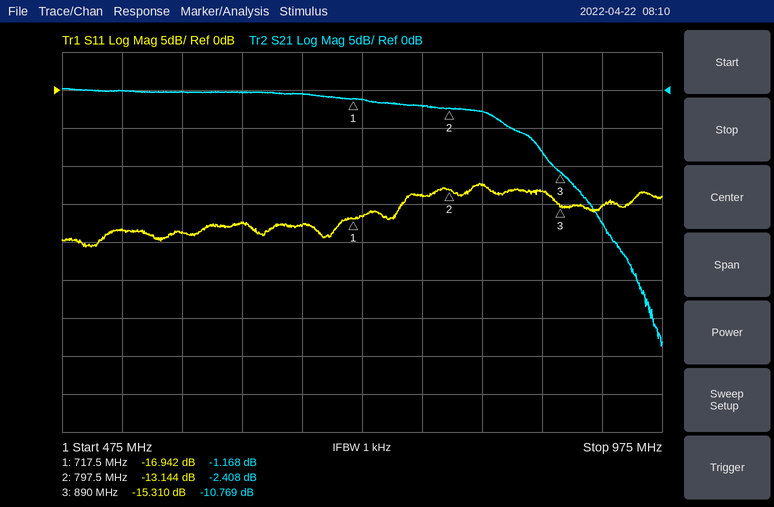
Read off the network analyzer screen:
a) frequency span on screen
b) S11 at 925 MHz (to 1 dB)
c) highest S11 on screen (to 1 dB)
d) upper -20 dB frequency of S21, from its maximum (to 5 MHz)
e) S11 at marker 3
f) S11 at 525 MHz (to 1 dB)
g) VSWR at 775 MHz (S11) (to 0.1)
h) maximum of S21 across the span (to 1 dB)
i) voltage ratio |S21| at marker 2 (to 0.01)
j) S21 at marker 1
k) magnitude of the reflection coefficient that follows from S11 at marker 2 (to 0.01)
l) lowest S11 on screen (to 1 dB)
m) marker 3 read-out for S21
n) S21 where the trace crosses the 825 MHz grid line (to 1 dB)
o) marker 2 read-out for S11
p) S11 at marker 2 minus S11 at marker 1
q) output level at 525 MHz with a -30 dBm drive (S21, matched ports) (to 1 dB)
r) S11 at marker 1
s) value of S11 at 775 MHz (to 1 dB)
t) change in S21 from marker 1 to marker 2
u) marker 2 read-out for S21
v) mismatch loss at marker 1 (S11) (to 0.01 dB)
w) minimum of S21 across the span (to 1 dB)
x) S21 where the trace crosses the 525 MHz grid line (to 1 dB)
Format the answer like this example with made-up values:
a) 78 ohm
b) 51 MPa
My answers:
a) 500 MHz
b) -15 dB
c) -12 dB
d) 935 MHz
e) -15.310 dB
f) -18 dB
g) 1.5
h) 0 dB
i) 0.76
j) -1.168 dB
k) 0.22
l) -21 dB
m) -10.769 dB
n) -3 dB
o) -13.144 dB
p) 3.798 dB
q) -30 dBm
r) -16.942 dB
s) -14 dB
t) -1.240 dB
u) -2.408 dB
v) 0.09 dB
w) -34 dB
x) 0 dB
